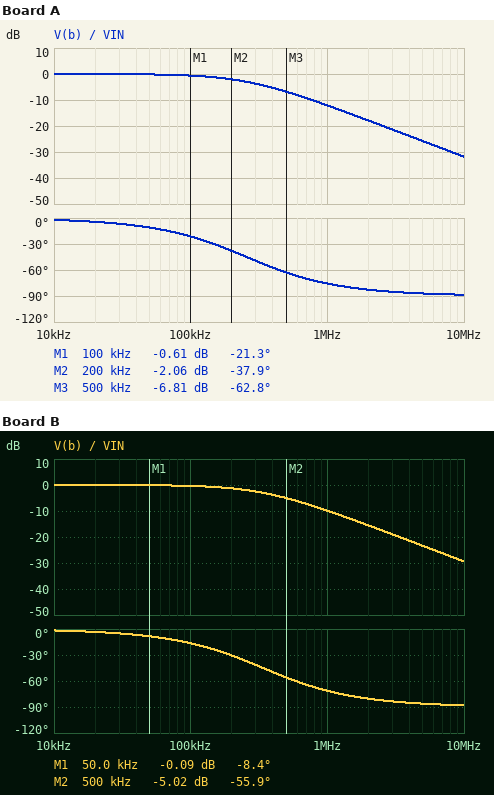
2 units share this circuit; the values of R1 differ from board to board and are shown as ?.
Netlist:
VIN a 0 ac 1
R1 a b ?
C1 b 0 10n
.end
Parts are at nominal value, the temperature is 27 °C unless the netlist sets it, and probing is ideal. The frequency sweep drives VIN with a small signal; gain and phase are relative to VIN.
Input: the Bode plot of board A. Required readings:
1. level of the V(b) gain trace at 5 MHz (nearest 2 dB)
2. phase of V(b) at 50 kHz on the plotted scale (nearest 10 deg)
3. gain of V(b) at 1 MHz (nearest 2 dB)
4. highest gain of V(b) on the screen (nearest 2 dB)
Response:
-26 dB
-10 deg
-12 dB
0 dB
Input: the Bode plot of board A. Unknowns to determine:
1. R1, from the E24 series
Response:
62 Ω
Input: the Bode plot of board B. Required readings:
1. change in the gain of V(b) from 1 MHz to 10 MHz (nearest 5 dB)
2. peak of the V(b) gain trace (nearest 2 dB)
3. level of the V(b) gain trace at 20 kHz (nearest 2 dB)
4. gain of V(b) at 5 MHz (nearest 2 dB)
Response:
-20 dB
0 dB
0 dB
-24 dB
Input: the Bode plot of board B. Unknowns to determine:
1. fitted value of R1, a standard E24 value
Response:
47 Ω
